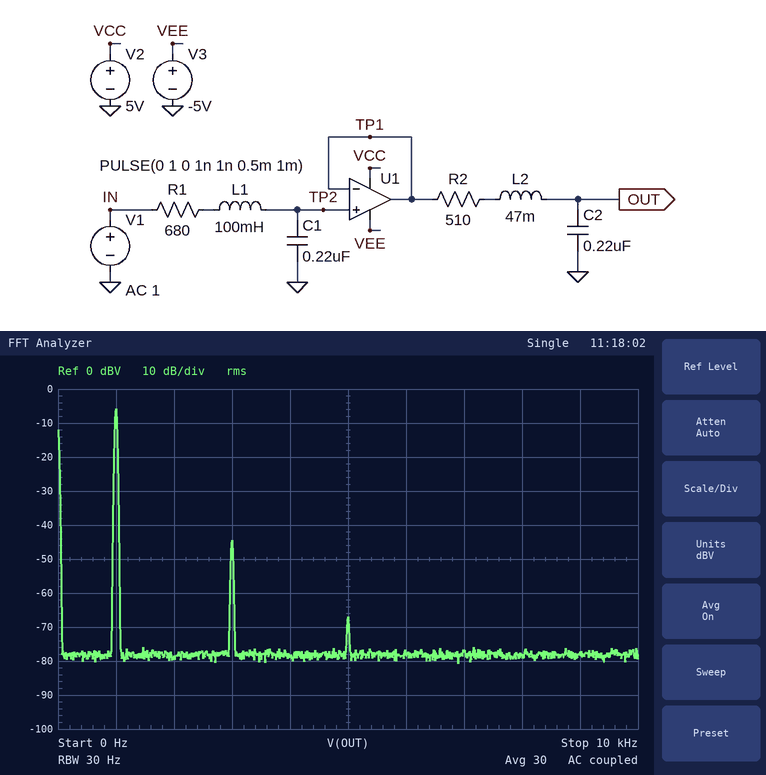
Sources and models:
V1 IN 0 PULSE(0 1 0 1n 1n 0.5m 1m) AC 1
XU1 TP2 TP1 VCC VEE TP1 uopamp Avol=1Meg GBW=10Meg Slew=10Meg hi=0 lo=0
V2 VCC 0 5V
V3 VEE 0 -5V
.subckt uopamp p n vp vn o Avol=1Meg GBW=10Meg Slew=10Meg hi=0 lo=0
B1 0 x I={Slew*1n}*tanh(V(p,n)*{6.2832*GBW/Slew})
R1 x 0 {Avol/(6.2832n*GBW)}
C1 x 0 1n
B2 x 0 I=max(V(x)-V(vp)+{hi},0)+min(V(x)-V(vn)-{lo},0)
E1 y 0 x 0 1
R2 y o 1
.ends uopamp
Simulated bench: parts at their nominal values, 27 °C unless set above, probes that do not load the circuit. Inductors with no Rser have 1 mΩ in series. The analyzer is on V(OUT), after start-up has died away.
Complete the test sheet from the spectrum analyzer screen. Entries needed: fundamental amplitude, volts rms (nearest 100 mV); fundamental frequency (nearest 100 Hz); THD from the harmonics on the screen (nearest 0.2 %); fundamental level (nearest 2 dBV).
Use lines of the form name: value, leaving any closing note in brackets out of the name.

fundamental amplitude, volts rms: 500 mV
fundamental frequency: 1.0 kHz
THD from the harmonics on the screen: 1.2 %
fundamental level: -6 dBV
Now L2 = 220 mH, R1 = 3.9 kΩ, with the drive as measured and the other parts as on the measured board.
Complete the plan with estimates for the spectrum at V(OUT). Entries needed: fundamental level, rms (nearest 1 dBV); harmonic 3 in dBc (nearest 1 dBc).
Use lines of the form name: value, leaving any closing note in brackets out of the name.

fundamental level, rms: -23 dBV
harmonic 3 in dBc: -43 dBc
